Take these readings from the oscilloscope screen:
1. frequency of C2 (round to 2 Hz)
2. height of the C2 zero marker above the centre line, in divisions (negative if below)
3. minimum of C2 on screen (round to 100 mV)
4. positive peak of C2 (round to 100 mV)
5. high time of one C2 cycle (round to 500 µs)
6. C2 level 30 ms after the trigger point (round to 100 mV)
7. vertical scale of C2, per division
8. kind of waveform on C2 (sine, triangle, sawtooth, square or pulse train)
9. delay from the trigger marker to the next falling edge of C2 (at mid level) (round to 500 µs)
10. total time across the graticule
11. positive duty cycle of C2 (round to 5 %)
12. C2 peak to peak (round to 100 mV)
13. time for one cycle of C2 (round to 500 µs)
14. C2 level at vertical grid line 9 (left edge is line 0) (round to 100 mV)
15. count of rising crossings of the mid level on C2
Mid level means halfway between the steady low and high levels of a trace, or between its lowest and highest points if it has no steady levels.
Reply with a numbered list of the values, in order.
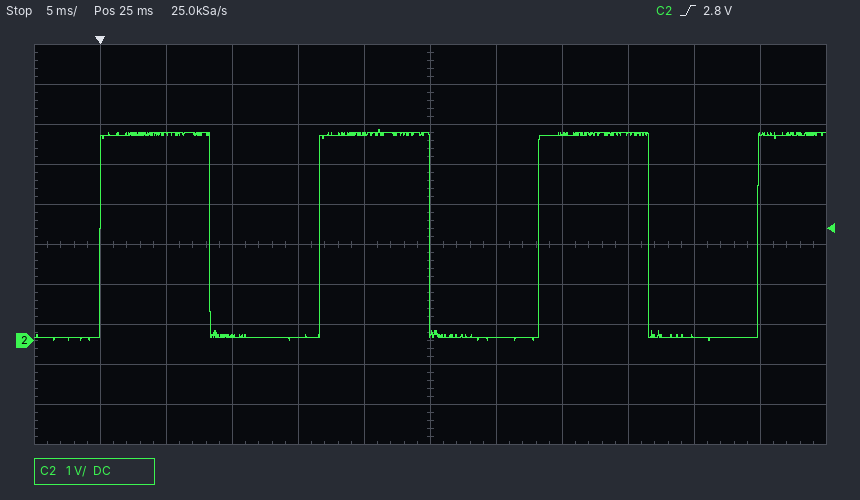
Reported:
1. 60 Hz
2. -2.4 div
3. 0.0 V
4. 5.3 V
5. 8.5 ms
6. 100 mV
7. 1 V
8. square
9. 8.5 ms
10. 60 ms
11. 50 %
12. 5.3 V
13. 16.5 ms
14. 5.2 V
15. 4
